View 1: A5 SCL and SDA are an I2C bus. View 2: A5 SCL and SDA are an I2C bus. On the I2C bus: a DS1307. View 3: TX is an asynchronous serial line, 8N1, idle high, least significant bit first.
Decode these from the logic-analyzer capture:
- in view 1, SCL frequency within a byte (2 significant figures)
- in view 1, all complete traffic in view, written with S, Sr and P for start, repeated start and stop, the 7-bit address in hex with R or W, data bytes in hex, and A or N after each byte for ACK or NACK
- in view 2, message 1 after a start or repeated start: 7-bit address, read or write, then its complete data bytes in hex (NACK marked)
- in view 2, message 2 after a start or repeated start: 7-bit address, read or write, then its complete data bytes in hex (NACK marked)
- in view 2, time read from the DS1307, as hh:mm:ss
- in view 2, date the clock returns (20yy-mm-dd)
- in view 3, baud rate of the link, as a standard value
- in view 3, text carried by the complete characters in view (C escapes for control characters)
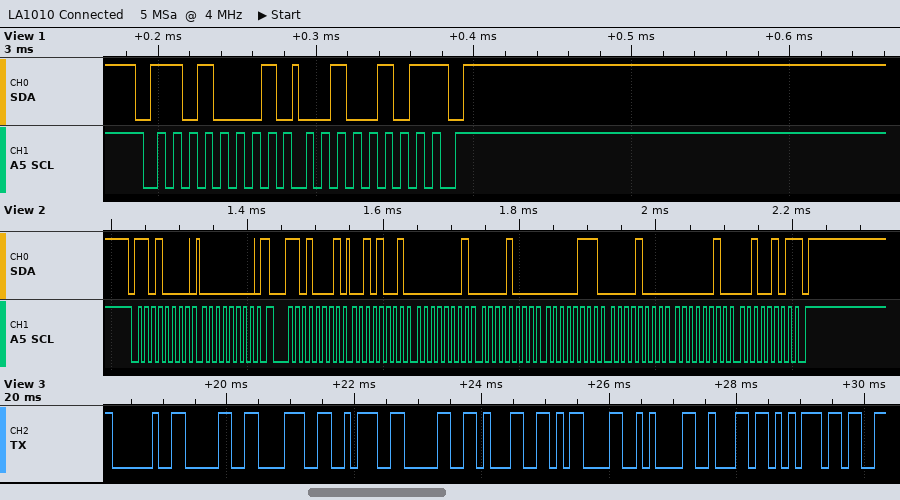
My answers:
100 kHz
S 68R A 25 N P
0x68 write: 00
0x68 read: 29 01 08 07 08 02 25 NACK
08:01:29
2025-02-08
9600 baud
" 08:01\r\nbu"
